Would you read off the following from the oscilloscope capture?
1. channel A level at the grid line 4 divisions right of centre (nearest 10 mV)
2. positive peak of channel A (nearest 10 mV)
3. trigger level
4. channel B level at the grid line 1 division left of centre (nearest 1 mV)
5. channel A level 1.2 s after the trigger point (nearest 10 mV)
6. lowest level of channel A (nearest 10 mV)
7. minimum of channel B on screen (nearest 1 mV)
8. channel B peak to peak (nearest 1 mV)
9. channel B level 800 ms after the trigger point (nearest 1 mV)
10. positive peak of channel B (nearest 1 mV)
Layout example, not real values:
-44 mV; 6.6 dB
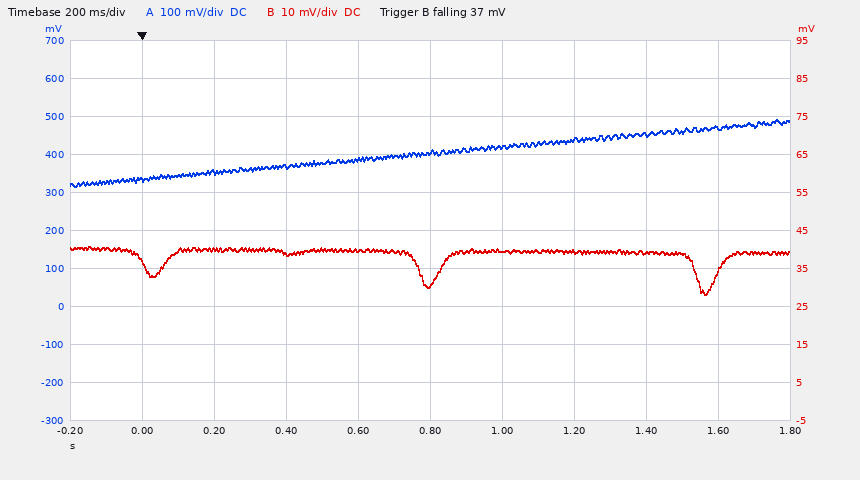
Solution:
470 mV; 490 mV; 37 mV; 40 mV; 440 mV; 320 mV; 28 mV; 13 mV; 31 mV; 41 mV
